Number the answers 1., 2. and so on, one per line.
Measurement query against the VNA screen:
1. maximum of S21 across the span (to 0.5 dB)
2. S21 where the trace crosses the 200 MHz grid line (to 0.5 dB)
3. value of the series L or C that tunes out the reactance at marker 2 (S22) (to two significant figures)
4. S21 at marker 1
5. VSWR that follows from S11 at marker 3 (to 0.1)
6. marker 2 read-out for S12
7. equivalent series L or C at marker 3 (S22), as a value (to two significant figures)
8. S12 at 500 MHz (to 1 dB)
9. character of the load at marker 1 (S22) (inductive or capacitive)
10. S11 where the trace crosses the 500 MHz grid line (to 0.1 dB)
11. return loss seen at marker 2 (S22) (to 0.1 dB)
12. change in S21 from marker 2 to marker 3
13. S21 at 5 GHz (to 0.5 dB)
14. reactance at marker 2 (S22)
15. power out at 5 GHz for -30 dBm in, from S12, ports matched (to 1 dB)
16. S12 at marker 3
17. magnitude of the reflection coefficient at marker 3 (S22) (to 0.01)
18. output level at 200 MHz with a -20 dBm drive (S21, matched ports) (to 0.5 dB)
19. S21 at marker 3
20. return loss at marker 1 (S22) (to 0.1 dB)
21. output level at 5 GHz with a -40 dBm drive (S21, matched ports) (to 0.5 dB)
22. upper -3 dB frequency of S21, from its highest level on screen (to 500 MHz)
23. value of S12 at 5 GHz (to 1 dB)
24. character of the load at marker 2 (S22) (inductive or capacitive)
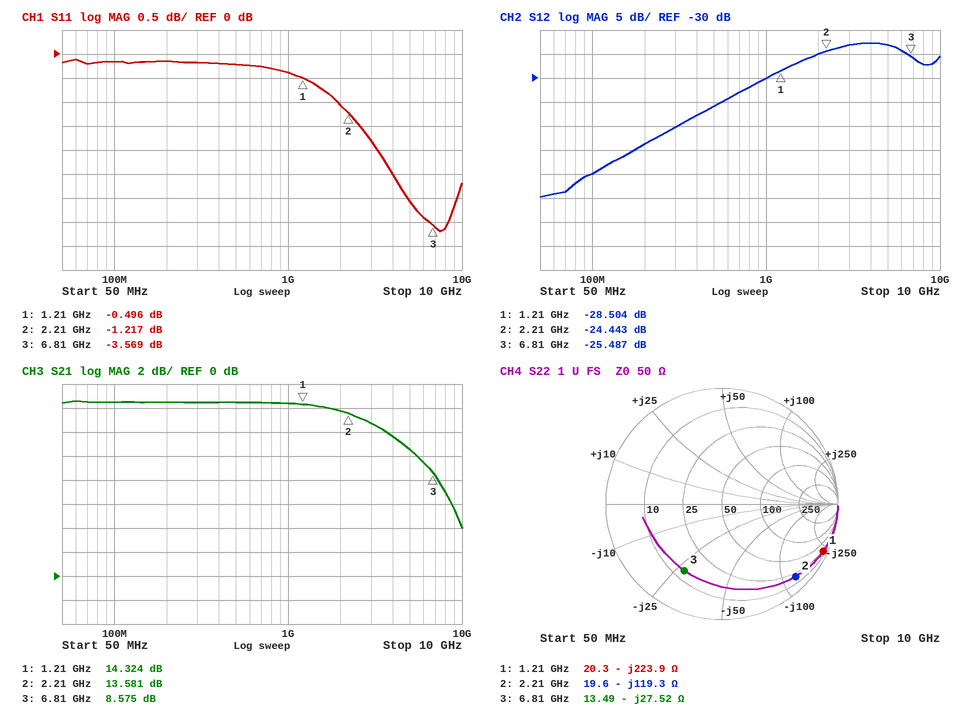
1. 14.5 dB
2. 14.5 dB
3. 8.6 nH
4. 14.324 dB
5. 4.9
6. -24.443 dB
7. 850 fF
8. -36 dB
9. capacitive
10. -0.2 dB
11. 1.0 dB
12. -5.006 dB
13. 10.5 dB
14. -119.3 Ω
15. -53 dBm
16. -25.487 dB
17. 0.66
18. -5.5 dBm
19. 8.575 dB
20. 0.3 dB
21. -29.5 dBm
22. 4.0 GHz
23. -23 dB
24. capacitive
